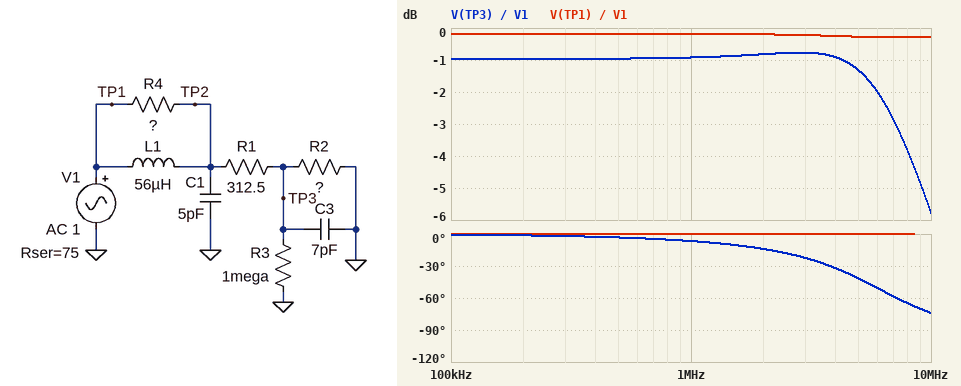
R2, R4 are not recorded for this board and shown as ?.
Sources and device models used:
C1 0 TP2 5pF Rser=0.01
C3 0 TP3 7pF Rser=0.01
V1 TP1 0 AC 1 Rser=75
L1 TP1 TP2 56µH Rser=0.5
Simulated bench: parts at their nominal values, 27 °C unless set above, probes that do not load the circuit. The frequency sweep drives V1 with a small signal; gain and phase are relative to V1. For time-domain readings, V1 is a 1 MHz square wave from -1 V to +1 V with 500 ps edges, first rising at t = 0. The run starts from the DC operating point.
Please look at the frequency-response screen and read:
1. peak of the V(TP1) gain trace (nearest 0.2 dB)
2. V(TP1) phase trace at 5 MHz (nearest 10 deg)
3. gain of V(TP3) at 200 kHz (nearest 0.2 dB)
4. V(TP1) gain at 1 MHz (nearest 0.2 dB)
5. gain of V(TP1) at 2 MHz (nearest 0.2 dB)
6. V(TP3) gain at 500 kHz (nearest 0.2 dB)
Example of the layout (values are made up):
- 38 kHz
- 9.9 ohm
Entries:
- -0.2 dB
- 0 deg
- -1.0 dB
- -0.2 dB
- -0.2 dB
- -1.0 dB
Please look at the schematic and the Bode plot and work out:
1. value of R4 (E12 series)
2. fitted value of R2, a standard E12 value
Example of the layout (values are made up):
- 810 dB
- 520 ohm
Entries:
- 2.7 kΩ
- 3.3 kΩ
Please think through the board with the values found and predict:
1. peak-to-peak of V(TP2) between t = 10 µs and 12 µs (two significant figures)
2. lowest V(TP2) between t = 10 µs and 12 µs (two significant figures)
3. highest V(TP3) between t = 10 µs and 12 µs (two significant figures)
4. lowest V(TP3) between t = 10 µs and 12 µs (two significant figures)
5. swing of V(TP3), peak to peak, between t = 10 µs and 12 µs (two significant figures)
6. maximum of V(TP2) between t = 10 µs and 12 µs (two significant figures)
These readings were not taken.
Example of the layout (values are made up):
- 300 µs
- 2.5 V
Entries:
- 2.2 V
- -1.1 V
- 1.0 V
- -1.0 V
- 2.0 V
- 1.1 V
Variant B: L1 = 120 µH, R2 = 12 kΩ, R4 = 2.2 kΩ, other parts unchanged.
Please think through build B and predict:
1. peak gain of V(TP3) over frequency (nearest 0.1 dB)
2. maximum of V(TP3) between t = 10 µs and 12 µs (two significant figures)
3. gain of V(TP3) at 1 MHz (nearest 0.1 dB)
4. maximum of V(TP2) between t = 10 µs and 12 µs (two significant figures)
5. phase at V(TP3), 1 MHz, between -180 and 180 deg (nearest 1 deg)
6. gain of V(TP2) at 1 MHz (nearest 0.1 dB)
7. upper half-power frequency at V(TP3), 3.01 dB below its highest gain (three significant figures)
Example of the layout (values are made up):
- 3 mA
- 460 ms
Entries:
- 0.4 dB
- 1.1 V
- 0 dB
- 1.2 V
- -5 deg
- 0.2 dB
- 6.71 MHz
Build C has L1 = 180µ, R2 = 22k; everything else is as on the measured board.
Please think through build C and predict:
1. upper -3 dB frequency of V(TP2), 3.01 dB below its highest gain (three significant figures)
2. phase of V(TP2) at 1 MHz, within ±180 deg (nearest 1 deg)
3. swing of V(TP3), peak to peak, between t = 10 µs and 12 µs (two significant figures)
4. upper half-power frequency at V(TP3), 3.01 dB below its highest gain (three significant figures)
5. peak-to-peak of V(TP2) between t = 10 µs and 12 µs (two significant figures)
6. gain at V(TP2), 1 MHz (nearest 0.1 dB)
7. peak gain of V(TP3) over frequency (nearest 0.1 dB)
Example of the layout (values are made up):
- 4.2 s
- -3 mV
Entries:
- 5.48 MHz
- -5 deg
- 2.4 V
- 5.46 MHz
- 2.5 V
- 0.4 dB
- 0.9 dB
